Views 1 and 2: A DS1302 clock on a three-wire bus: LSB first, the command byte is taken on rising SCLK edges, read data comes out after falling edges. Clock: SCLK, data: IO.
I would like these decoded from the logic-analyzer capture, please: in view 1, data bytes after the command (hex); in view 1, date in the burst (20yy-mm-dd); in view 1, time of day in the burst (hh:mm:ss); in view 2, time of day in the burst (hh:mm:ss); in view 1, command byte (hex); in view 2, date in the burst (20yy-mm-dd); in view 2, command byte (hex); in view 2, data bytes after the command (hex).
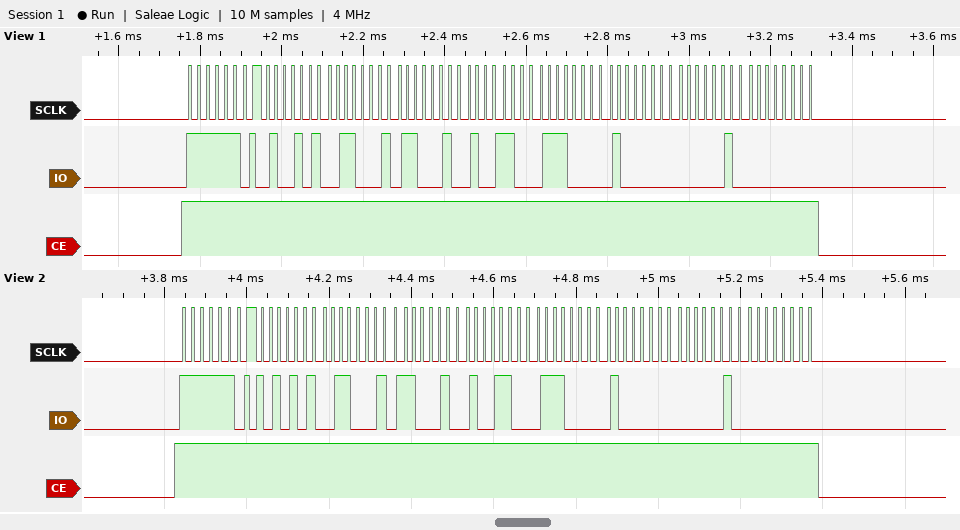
52 46 23 19 07 01 20 00
2020-07-19
23:46:52
23:46:55
0xBF
2020-07-19
0xBF
55 46 23 19 07 01 20 00
